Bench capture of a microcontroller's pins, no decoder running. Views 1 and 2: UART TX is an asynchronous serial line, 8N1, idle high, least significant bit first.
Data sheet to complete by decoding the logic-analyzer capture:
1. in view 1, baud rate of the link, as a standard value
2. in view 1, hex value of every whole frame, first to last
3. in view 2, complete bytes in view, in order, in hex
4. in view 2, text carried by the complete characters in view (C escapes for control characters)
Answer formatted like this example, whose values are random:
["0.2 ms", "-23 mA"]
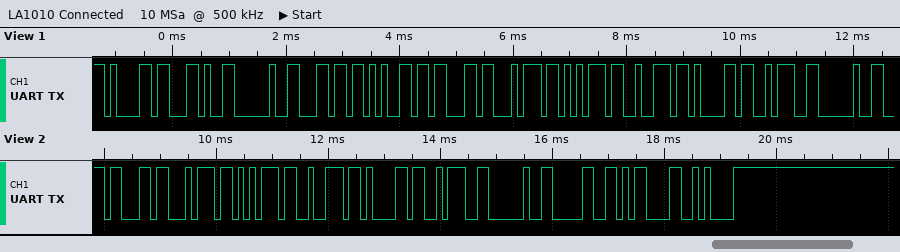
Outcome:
["9600 baud", "61 2C 20 6C 65 63 74 75 72 61 3A 20", "63 74 75 72 61 3A 20 30 0D 0A", "\"ctura: 0\\r\\n\""]
